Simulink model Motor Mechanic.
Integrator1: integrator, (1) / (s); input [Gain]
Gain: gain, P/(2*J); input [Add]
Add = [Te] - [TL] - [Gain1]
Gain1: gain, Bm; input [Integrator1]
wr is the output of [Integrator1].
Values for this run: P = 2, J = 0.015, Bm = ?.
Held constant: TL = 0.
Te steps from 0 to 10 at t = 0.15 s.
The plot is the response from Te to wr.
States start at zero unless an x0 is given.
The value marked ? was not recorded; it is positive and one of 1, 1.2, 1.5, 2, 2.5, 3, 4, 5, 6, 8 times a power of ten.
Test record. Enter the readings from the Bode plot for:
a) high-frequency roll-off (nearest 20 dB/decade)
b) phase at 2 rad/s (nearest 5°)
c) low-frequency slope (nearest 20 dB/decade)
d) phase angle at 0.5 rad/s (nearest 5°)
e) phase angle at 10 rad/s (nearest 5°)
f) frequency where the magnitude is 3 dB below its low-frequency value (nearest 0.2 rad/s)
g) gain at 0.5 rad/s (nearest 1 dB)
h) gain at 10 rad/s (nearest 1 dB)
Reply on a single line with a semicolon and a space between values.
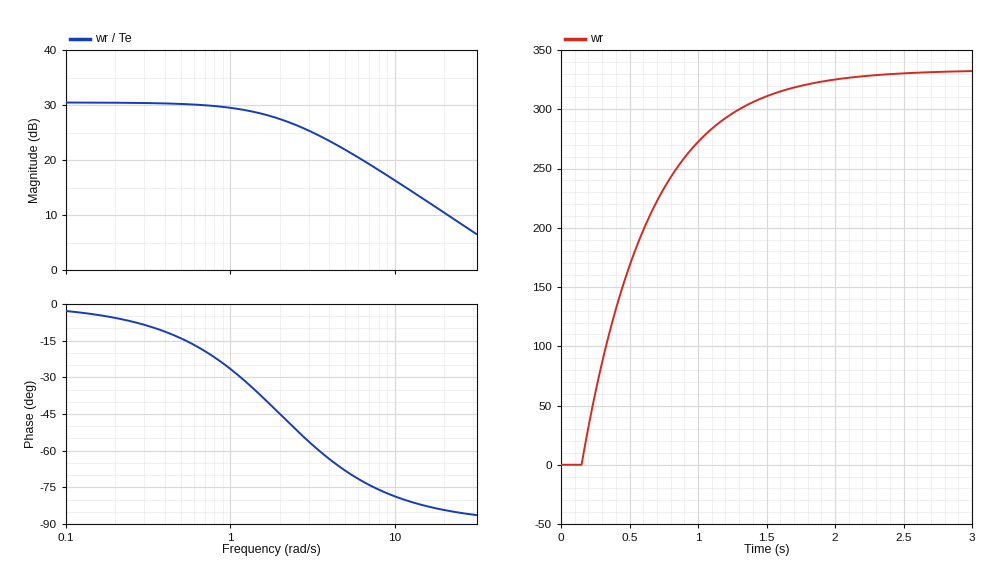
-20 dB/decade; -45°; 0 dB/decade; -15°; -80°; 2.0 rad/s; 30 dB; 16 dB
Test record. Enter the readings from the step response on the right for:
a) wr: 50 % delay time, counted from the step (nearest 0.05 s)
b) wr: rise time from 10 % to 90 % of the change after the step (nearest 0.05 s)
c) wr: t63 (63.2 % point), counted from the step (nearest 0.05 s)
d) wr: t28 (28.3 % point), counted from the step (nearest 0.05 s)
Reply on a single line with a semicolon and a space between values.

0.35 s; 1.10 s; 0.50 s; 0.15 s
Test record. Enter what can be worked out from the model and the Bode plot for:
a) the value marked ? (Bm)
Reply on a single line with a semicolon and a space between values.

0.03
